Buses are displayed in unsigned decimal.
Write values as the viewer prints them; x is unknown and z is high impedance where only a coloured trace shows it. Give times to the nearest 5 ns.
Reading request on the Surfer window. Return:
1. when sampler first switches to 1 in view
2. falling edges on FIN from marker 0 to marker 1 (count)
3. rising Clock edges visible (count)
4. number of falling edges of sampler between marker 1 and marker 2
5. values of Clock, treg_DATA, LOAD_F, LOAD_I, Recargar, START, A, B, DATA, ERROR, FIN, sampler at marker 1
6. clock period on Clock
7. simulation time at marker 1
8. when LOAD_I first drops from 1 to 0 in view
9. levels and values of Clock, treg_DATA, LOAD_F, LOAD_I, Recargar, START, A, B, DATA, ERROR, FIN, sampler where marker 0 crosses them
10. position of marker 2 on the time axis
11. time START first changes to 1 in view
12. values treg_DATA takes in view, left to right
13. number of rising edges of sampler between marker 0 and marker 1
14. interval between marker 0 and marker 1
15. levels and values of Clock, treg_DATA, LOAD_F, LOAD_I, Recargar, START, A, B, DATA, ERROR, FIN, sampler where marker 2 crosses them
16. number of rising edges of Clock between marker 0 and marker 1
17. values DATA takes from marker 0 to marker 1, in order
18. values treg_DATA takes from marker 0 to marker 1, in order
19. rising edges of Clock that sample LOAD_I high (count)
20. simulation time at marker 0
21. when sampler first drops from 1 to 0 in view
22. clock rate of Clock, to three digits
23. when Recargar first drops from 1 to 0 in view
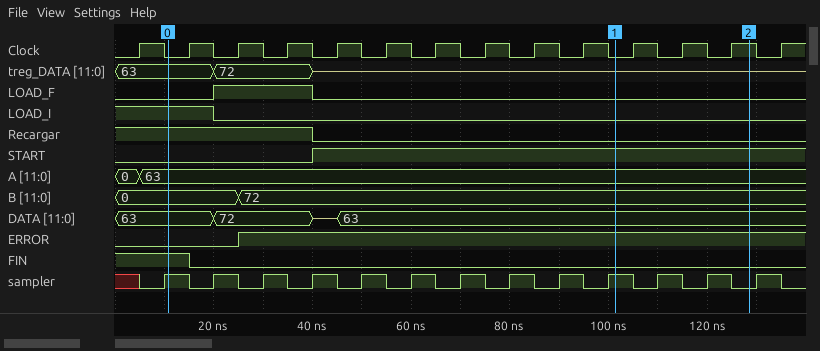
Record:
10 ns
1
14
3
Clock=0, treg_DATA=z, LOAD_F=0, LOAD_I=0, Recargar=0, START=1, A=63, B=72, DATA=63, ERROR=1, FIN=0, sampler=1
10 ns
100 ns
20 ns
Clock=0, treg_DATA=63, LOAD_F=0, LOAD_I=1, Recargar=1, START=0, A=63, B=0, DATA=63, ERROR=0, FIN=1, sampler=1
130 ns
40 ns
63, 72, z
9
90 ns
Clock=1, treg_DATA=z, LOAD_F=0, LOAD_I=0, Recargar=0, START=1, A=63, B=72, DATA=63, ERROR=1, FIN=0, sampler=0
9
63, 72, z, 63
63, 72, z
2
10 ns
15 ns
100 MHz
40 ns
